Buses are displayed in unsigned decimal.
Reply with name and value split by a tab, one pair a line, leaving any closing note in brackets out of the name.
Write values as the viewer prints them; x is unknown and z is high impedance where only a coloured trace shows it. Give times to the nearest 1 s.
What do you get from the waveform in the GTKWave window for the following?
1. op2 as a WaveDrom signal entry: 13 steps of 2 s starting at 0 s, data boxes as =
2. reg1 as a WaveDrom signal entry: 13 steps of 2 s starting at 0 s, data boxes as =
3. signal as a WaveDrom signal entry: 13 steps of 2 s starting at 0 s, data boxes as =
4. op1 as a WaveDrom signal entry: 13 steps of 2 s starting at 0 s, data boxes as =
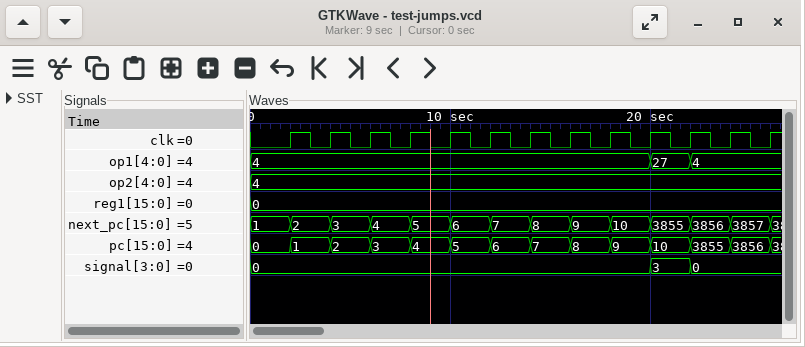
op2 as a WaveDrom signal entry: 13 steps of 2 s starting at 0 s, data boxes as =	{name: 'op2', wave: '=............', data: '4'}
reg1 as a WaveDrom signal entry: 13 steps of 2 s starting at 0 s, data boxes as =	{name: 'reg1', wave: '=............', data: '0'}
signal as a WaveDrom signal entry: 13 steps of 2 s starting at 0 s, data boxes as =	{name: 'signal', wave: '=.........==.', data: '0 3 0'}
op1 as a WaveDrom signal entry: 13 steps of 2 s starting at 0 s, data boxes as =	{name: 'op1', wave: '=.........==.', data: '4 27 4'}
